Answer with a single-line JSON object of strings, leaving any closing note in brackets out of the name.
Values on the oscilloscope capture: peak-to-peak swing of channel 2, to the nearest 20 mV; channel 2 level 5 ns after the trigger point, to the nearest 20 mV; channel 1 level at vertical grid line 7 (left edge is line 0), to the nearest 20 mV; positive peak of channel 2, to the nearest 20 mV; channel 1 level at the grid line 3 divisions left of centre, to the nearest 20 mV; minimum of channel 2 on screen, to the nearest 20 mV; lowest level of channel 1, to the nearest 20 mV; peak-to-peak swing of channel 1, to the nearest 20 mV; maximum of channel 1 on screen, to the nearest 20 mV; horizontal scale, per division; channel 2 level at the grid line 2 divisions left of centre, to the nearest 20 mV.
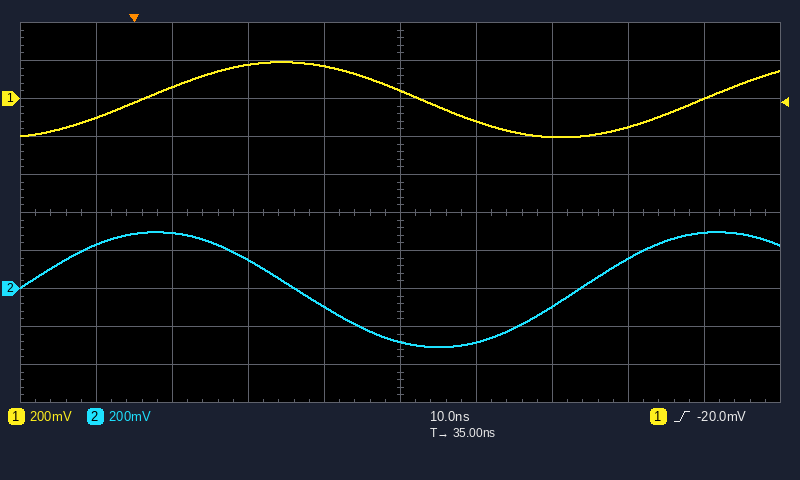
{"peak-to-peak swing of channel 2, to the nearest 20 mV": "600 mV", "channel 2 level 5 ns after the trigger point, to the nearest 20 mV": "300 mV", "channel 1 level at vertical grid line 7 (left edge is line 0), to the nearest 20 mV": "-200 mV", "positive peak of channel 2, to the nearest 20 mV": "300 mV", "channel 1 level at the grid line 3 divisions left of centre, to the nearest 20 mV": "60 mV", "minimum of channel 2 on screen, to the nearest 20 mV": "-300 mV", "lowest level of channel 1, to the nearest 20 mV": "-200 mV", "peak-to-peak swing of channel 1, to the nearest 20 mV": "400 mV", "maximum of channel 1 on screen, to the nearest 20 mV": "200 mV", "horizontal scale, per division": "10 ns", "channel 2 level at the grid line 2 divisions left of centre, to the nearest 20 mV": "160 mV"}
